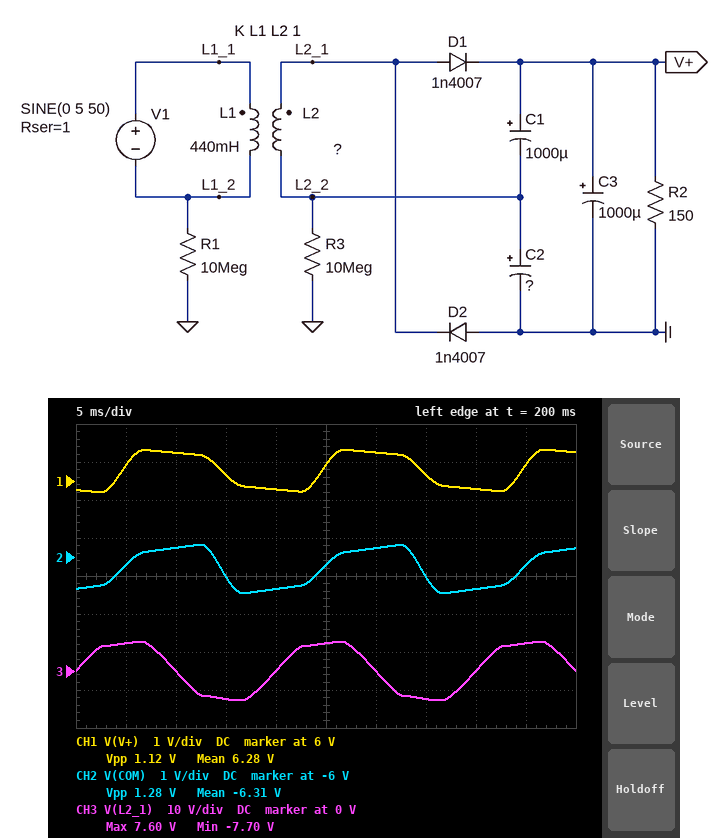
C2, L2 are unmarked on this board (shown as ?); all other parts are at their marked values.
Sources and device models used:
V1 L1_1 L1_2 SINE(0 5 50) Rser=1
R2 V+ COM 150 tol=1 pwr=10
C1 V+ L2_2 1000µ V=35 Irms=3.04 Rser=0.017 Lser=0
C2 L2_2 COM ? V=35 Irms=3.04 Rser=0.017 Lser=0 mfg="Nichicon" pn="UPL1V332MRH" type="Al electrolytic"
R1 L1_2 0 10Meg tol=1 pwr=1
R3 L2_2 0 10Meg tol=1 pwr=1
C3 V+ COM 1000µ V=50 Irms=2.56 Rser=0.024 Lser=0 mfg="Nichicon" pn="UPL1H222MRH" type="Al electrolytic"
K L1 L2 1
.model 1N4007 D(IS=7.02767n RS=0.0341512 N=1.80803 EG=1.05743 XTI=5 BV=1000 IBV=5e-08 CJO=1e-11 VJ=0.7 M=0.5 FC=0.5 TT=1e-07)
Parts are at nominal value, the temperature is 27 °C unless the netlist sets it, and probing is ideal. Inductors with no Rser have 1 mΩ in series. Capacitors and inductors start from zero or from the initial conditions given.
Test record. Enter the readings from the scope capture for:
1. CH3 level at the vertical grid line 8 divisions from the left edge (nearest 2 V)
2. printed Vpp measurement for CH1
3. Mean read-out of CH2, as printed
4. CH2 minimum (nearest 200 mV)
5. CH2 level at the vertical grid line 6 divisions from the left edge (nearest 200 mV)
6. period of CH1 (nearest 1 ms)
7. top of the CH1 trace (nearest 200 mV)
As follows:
0 V
1.12 V
-6.31 V
-7.0 V
-5.8 V
20 ms
6.8 V
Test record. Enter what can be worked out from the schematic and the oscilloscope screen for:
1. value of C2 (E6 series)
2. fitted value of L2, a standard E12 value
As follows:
680 µF
1.5 H
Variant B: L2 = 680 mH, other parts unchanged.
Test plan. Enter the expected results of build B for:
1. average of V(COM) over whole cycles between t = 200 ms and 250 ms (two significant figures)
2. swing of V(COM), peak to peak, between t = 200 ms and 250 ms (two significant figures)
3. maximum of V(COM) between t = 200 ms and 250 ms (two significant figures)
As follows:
-4.5 V
920 mV
-4.0 V
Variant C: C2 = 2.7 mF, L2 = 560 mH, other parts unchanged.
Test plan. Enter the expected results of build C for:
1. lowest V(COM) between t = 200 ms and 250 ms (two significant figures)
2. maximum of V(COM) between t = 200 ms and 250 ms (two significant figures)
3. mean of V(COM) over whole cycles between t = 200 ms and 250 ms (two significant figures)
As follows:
-4.3 V
-4.0 V
-4.2 V
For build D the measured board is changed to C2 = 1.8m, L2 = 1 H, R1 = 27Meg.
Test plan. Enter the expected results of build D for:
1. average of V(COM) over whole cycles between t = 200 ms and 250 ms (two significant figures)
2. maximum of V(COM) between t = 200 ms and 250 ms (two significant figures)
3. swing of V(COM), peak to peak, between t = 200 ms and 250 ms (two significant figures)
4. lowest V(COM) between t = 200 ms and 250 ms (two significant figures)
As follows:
-5.4 V
-5.1 V
570 mV
-5.7 V
